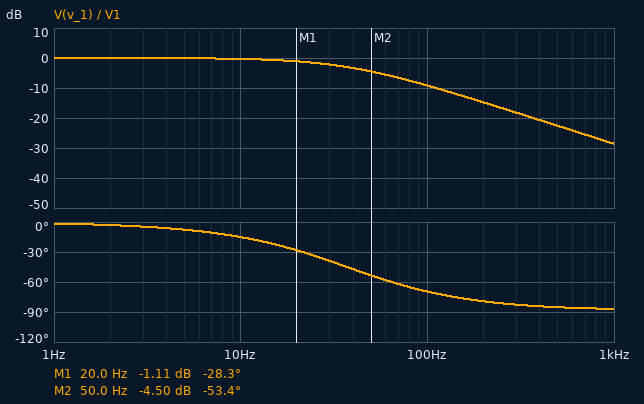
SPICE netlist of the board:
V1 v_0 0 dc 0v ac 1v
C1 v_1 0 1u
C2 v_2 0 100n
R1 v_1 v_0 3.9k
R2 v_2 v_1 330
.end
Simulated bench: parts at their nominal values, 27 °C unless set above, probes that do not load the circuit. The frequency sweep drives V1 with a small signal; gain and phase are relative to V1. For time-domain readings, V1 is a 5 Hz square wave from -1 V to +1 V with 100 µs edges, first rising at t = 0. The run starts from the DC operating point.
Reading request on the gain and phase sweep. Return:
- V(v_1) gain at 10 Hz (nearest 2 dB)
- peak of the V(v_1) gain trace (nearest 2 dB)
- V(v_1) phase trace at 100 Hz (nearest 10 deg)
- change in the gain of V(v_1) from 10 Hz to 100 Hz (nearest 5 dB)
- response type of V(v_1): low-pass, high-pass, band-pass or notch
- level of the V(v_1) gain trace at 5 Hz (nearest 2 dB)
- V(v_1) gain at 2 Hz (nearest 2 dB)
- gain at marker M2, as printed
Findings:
0 dB
0 dB
-70 deg
-10 dB
low-pass
0 dB
0 dB
-4.50 dB
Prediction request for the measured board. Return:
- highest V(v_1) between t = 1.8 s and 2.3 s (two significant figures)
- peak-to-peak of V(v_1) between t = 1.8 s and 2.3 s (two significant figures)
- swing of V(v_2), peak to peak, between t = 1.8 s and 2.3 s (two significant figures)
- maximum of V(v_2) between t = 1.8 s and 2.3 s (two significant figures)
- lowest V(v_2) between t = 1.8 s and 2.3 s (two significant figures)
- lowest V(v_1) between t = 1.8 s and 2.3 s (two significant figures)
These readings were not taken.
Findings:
1.0 V
2.0 V
2.0 V
1.0 V
-1.0 V
-1.0 V
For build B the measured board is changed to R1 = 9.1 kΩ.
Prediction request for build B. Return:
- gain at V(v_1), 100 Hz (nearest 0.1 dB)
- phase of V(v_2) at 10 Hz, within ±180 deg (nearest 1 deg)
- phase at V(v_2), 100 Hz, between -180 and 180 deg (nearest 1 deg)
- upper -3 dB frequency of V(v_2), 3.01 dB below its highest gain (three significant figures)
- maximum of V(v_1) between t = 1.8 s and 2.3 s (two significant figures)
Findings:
-16.1 dB
-32 deg
-82 deg
15.9 Hz
1.0 V
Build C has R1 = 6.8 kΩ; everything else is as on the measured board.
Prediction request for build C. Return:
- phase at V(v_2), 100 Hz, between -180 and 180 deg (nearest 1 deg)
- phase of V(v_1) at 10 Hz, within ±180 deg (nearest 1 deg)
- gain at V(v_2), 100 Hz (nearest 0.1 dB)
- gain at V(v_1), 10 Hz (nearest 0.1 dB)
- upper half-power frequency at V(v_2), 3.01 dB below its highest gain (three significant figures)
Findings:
-79 deg
-25 deg
-13.6 dB
-0.9 dB
21.3 Hz
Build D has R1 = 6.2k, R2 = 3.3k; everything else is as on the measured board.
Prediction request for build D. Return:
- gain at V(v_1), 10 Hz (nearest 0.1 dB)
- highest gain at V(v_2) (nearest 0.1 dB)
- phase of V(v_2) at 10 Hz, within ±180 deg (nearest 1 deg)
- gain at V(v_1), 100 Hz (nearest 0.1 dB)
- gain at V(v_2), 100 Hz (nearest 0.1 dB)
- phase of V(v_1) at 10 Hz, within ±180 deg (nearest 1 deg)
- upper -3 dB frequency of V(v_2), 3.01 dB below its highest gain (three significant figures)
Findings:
-0.7 dB
0 dB
-24 deg
-12.9 dB
-13.1 dB
-23 deg
23.2 Hz
